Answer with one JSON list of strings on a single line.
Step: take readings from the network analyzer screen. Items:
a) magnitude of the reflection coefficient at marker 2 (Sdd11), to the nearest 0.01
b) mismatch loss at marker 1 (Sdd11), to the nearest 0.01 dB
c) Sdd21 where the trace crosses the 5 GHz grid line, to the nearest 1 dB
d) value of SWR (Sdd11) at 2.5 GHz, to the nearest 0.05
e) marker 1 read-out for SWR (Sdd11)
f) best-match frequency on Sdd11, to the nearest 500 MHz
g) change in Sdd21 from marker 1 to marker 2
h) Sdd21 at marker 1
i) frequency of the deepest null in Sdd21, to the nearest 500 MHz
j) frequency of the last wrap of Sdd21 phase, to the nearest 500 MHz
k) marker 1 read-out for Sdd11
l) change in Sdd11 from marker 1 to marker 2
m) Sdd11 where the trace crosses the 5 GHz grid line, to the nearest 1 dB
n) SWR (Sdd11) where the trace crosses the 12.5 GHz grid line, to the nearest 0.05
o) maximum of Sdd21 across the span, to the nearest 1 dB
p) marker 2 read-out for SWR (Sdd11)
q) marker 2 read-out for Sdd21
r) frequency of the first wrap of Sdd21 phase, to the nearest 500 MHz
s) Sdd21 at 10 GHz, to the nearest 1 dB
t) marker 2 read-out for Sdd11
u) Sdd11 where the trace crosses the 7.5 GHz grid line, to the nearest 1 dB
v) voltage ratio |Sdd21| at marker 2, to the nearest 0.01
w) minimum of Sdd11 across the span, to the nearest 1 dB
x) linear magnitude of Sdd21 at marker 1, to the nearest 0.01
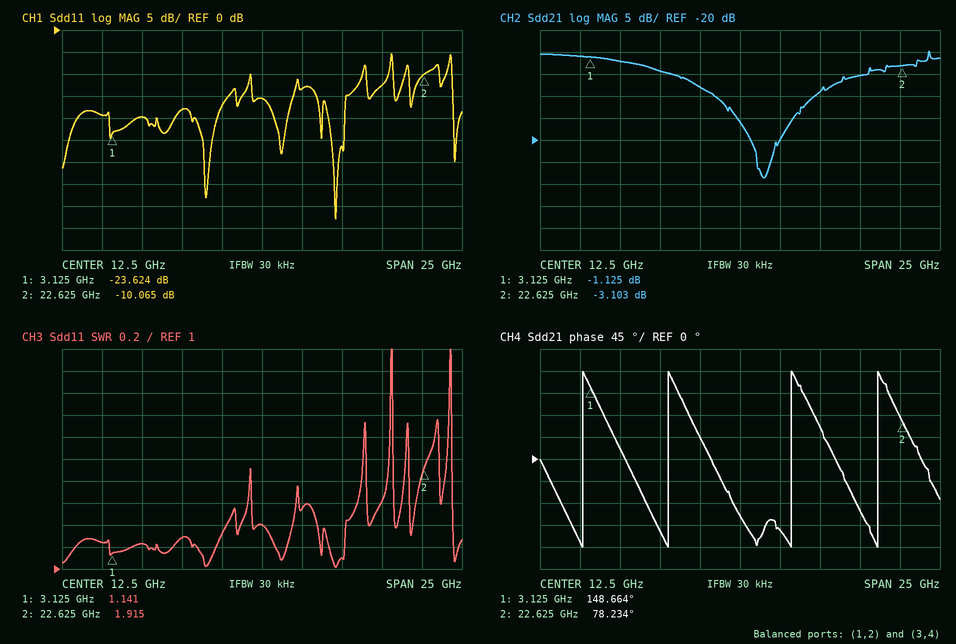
["0.31", "0.02 dB", "-2 dB", "1.25", "1.141", "17.0 GHz", "-1.978 dB", "-1.125 dB", "14.0 GHz", "21.0 GHz", "-23.624 dB", "13.559 dB", "-20 dB", "1.40", "0 dB", "1.915", "-3.103 dB", "2.5 GHz", "-8 dB", "-10.065 dB", "-18 dB", "0.70", "-43 dB", "0.88"]
